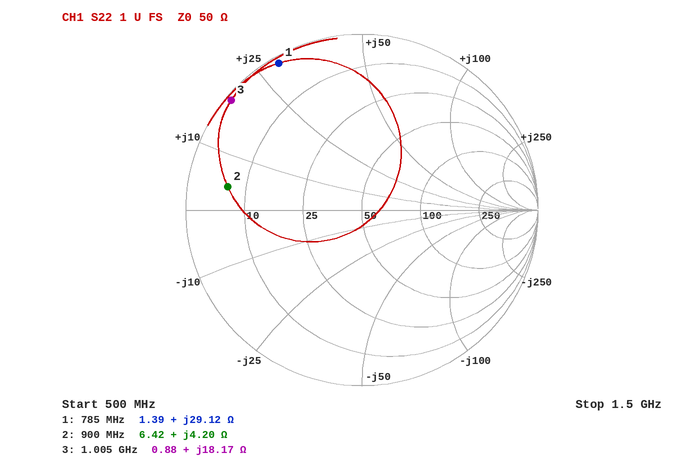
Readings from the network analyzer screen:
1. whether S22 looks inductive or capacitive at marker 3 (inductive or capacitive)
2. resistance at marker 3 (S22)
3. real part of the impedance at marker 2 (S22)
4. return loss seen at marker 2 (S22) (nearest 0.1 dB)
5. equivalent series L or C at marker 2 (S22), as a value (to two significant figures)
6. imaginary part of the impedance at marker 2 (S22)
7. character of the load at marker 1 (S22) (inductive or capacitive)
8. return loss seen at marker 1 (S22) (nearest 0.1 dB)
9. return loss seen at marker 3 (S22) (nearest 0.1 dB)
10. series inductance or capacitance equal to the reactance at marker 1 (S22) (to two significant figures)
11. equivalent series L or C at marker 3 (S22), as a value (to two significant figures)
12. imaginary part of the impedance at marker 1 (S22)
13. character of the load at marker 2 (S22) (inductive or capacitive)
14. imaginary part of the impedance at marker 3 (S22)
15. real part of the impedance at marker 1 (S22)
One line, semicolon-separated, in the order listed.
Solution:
inductive; 0.88 Ω; 6.42 Ω; 2.2 dB; 740 pH; +4.20 Ω; inductive; 0.4 dB; 0.3 dB; 5.9 nH; 2.9 nH; +29.12 Ω; inductive; +18.17 Ω; 1.39 Ω
